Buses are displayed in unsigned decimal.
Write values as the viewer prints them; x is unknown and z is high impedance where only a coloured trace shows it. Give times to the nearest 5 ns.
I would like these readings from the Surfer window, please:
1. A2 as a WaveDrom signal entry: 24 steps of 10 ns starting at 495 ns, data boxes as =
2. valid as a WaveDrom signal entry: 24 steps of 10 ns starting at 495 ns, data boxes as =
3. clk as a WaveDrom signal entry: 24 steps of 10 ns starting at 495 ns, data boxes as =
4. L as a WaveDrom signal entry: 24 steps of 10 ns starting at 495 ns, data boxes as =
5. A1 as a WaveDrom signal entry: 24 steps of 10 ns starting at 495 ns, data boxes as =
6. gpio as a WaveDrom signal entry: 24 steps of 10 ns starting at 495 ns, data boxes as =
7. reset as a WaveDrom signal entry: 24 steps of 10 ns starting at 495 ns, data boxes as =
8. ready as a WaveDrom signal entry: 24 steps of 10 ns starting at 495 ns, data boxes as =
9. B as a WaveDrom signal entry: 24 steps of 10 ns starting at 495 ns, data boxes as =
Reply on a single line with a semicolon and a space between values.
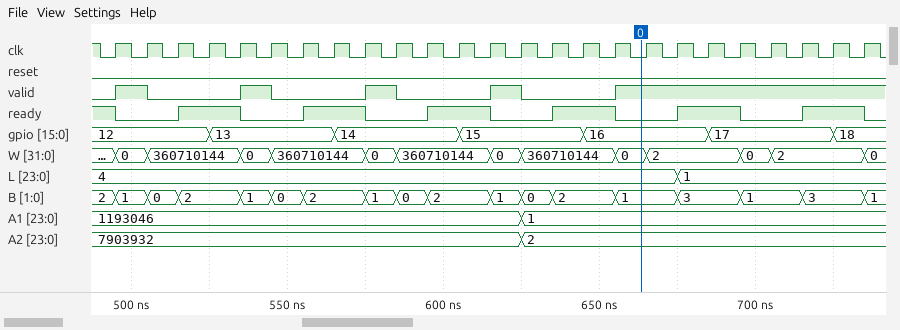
{name: 'A2', wave: '=............=..........', data: '7903932 2'}; {name: 'valid', wave: '10..10..10..10..1.......'}; {name: 'clk', wave: 'p.......................'}; {name: 'L', wave: '=.................=.....', data: '4 1'}; {name: 'A1', wave: '=............=..........', data: '1193046 1'}; {name: 'gpio', wave: '=..=...=...=...=...=...=', data: '12 13 14 15 16 17 18'}; {name: 'reset', wave: '0.......................'}; {name: 'ready', wave: '0.1.0.1.0.1.0.1.0.1.0.1.'}; {name: 'B', wave: '===.===.===.===.=.=.=.=.', data: '1 0 2 1 0 2 1 0 2 1 0 2 1 3 1 3'}
